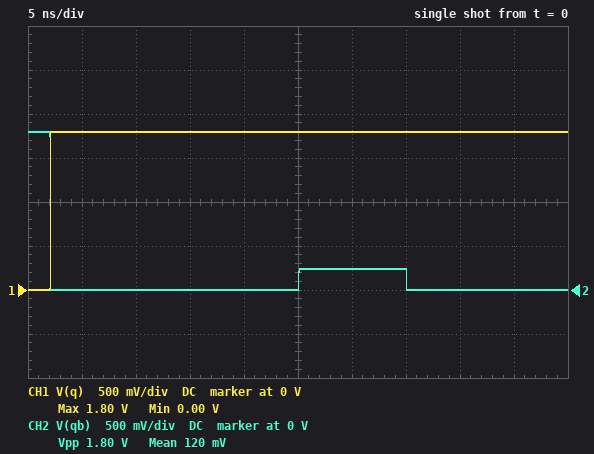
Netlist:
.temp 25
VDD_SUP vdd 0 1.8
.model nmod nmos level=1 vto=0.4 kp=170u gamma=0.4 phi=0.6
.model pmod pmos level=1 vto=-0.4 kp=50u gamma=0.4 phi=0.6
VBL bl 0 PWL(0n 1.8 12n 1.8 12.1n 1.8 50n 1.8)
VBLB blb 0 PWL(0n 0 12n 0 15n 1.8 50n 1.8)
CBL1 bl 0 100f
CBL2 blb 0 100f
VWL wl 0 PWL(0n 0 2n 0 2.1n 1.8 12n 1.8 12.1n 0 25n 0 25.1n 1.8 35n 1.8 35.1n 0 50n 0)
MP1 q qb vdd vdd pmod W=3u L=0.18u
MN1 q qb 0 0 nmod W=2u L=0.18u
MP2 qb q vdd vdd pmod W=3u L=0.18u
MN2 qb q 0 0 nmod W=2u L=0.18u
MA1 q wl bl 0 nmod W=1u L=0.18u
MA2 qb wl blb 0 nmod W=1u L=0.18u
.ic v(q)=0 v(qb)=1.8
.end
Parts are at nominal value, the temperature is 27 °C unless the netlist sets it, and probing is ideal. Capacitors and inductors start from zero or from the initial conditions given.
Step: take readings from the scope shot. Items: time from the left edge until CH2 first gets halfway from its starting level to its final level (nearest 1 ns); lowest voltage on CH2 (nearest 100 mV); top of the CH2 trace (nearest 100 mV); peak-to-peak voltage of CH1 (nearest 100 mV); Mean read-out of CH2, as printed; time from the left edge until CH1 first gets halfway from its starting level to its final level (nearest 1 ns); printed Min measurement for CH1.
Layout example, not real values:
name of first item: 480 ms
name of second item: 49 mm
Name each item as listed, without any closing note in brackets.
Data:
time from the left edge until CH2 first gets halfway from its starting level to its final level: 2 ns
lowest voltage on CH2: 0 V
top of the CH2 trace: 1.8 V
peak-to-peak voltage of CH1: 1.8 V
Mean read-out of CH2, as printed: 120 mV
time from the left edge until CH1 first gets halfway from its starting level to its final level: 2 ns
printed Min measurement for CH1: 0.00 V
